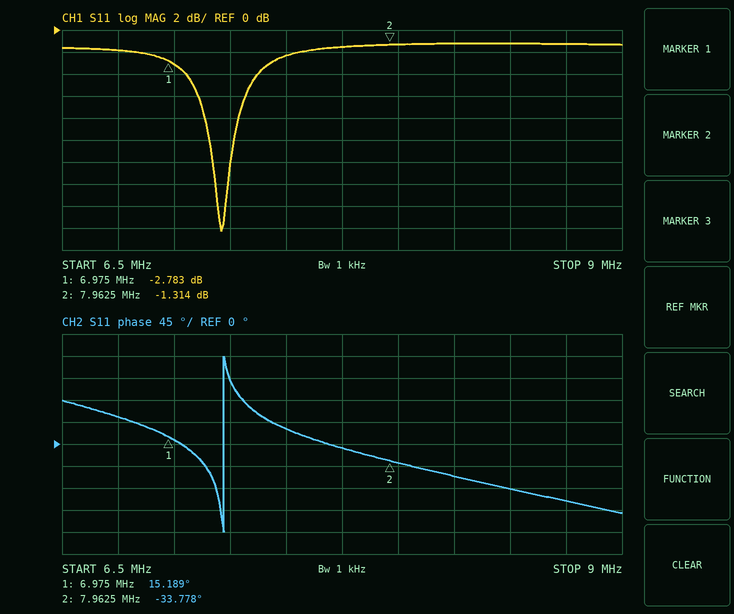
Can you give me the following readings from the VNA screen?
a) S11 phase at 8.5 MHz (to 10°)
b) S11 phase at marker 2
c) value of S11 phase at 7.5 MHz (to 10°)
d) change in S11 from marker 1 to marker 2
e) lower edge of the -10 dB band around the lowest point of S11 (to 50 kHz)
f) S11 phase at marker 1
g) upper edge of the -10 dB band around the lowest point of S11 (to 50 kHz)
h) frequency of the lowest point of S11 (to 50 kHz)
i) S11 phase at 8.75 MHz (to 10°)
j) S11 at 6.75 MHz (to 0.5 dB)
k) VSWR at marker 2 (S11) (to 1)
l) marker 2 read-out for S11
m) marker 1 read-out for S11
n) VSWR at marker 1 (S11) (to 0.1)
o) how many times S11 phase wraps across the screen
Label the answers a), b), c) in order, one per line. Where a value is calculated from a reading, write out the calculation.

a) -90°
b) -33.778°
c) 30°
d) -1.314 − (-2.783) = 1.469 dB
e) 7.15 MHz
f) 15.189°
g) 7.25 MHz
h) 7.20 MHz
i) -120°
j) -2.0 dB
k) (1 + 0.8596)/(1 − 0.8596) ≈ 13
l) -1.314 dB
m) -2.783 dB
n) (1 + 0.7259)/(1 − 0.7259) ≈ 6.3
o) 1
